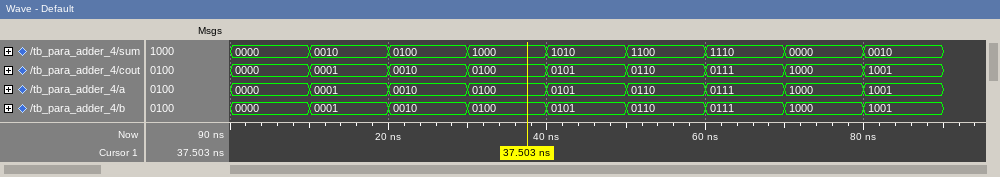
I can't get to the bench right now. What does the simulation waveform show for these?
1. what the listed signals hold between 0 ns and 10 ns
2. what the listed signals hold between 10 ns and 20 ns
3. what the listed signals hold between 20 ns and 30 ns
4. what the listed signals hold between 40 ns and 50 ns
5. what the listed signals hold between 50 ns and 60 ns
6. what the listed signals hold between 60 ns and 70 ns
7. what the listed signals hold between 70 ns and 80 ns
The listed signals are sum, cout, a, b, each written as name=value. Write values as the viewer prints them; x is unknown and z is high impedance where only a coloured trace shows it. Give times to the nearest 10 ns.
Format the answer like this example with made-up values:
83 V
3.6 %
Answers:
sum=0000, cout=0000, a=0000, b=0000
sum=0010, cout=0001, a=0001, b=0001
sum=0100, cout=0010, a=0010, b=0010
sum=1010, cout=0101, a=0101, b=0101
sum=1100, cout=0110, a=0110, b=0110
sum=1110, cout=0111, a=0111, b=0111
sum=0000, cout=1000, a=1000, b=1000
